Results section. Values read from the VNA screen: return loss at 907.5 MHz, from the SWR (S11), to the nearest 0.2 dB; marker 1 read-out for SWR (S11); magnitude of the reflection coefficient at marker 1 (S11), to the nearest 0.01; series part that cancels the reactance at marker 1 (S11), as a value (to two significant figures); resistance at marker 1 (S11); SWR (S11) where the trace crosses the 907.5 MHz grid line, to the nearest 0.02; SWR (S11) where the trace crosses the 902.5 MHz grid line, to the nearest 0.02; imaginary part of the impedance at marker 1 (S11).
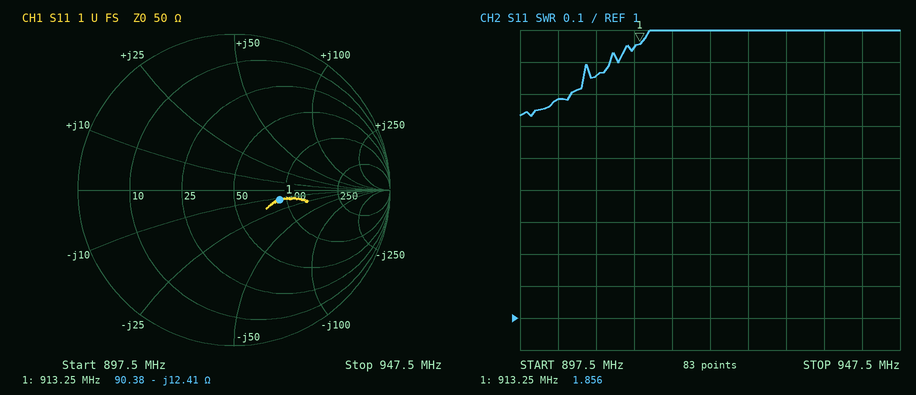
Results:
11.2 dB
1.856
0.30
2.2 nH
90.38 Ω
1.76
1.68
-12.41 Ω
